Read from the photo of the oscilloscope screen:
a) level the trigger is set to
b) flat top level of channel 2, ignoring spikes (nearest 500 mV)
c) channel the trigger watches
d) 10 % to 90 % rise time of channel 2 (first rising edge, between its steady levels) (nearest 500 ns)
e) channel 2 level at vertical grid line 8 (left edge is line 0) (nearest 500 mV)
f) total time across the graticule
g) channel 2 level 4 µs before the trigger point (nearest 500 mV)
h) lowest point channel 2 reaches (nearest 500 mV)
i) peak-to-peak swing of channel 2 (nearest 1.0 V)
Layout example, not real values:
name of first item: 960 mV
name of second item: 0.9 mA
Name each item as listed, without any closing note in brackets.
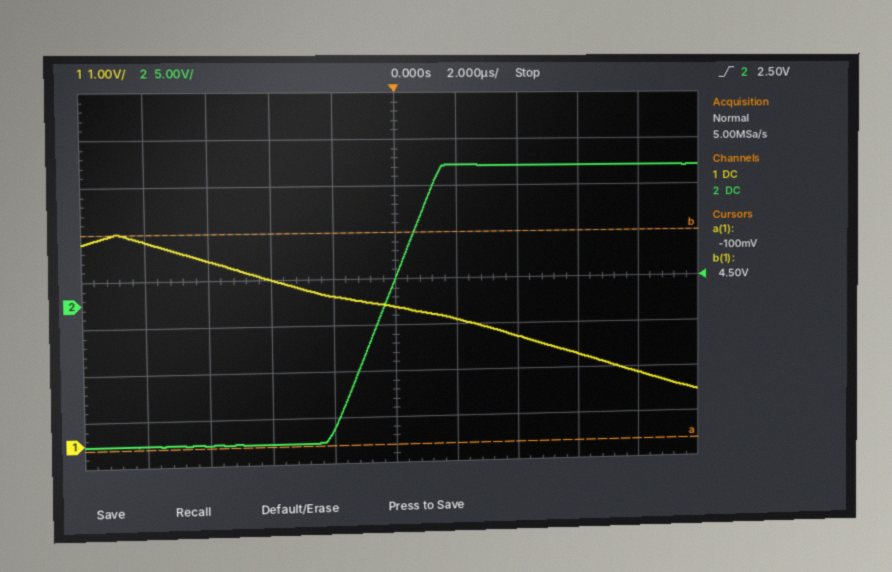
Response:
level the trigger is set to: 2.50 V
flat top level of channel 2, ignoring spikes: 14.5 V
channel the trigger watches: channel 2
10 % to 90 % rise time of channel 2 (first rising edge, between its steady levels): 3.0 µs
channel 2 level at vertical grid line 8 (left edge is line 0): 14.5 V
total time across the graticule: 20 µs
channel 2 level 4 µs before the trigger point: -15.0 V
lowest point channel 2 reaches: -15.0 V
peak-to-peak swing of channel 2: 30.0 V
